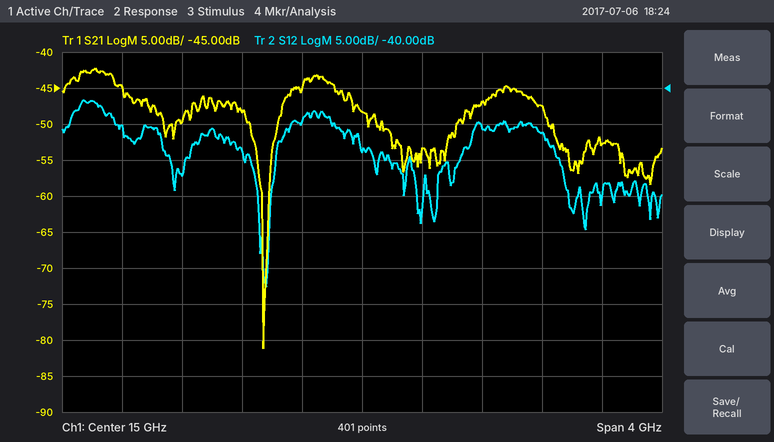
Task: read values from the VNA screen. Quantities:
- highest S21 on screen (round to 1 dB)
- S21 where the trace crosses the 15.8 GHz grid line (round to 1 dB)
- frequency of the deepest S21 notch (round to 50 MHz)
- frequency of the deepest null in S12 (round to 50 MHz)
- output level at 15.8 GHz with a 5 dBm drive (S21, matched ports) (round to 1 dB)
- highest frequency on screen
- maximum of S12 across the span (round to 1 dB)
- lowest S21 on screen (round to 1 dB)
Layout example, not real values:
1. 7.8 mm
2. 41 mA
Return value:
1. -42 dB
2. -47 dB
3. 14.35 GHz
4. 14.35 GHz
5. -42 dBm
6. 17 GHz
7. -42 dB
8. -81 dB
